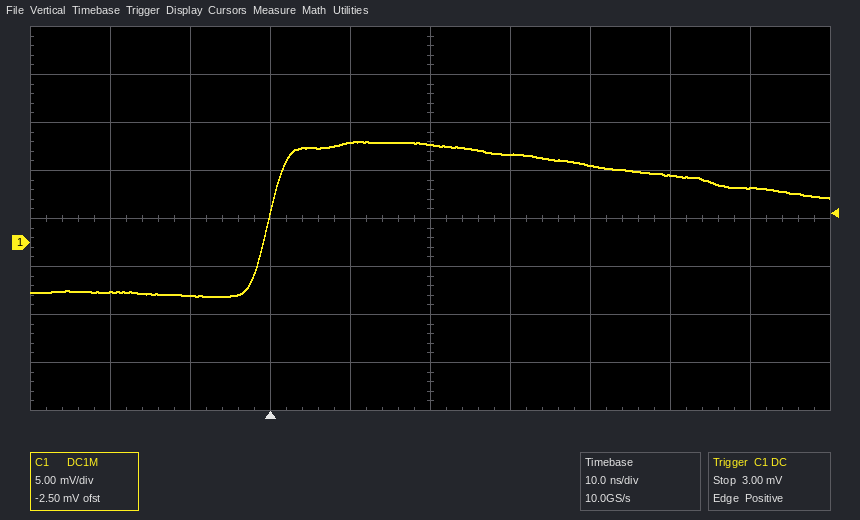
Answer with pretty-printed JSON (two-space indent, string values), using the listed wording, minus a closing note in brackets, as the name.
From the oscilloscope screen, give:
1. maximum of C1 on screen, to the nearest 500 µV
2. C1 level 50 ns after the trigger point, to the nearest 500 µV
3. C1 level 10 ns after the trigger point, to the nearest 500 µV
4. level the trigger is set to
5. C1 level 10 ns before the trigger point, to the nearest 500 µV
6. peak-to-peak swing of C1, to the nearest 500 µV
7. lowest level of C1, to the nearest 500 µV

{
  "maximum of C1 on screen, to the nearest 500 µV": "10.5 mV",
  "C1 level 50 ns after the trigger point, to the nearest 500 µV": "7.0 mV",
  "C1 level 10 ns after the trigger point, to the nearest 500 µV": "10.5 mV",
  "level the trigger is set to": "3.00 mV",
  "C1 level 10 ns before the trigger point, to the nearest 500 µV": "-5.5 mV",
  "peak-to-peak swing of C1, to the nearest 500 µV": "16.0 mV",
  "lowest level of C1, to the nearest 500 µV": "-5.5 mV"
}
